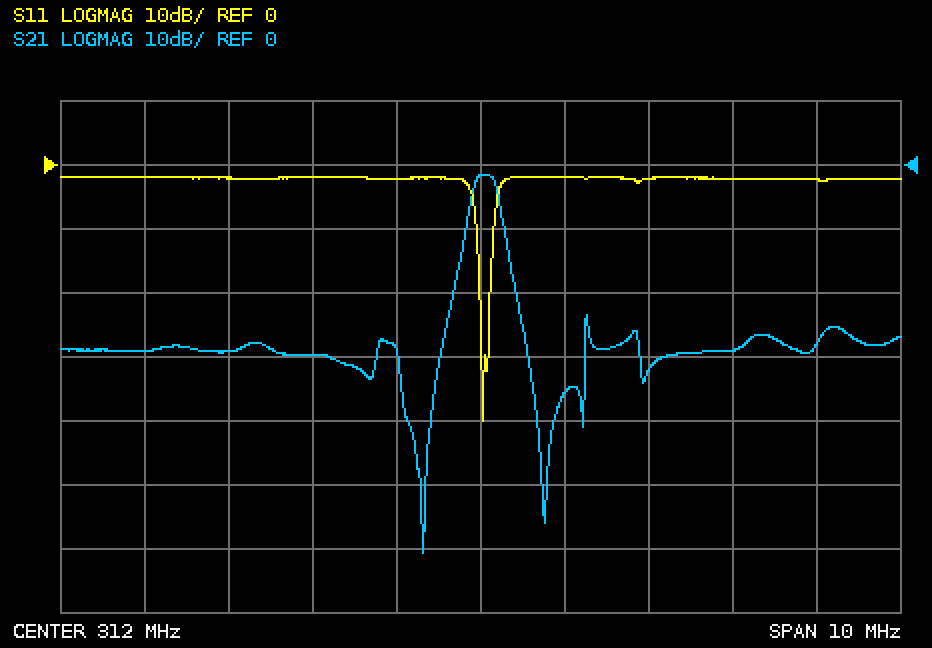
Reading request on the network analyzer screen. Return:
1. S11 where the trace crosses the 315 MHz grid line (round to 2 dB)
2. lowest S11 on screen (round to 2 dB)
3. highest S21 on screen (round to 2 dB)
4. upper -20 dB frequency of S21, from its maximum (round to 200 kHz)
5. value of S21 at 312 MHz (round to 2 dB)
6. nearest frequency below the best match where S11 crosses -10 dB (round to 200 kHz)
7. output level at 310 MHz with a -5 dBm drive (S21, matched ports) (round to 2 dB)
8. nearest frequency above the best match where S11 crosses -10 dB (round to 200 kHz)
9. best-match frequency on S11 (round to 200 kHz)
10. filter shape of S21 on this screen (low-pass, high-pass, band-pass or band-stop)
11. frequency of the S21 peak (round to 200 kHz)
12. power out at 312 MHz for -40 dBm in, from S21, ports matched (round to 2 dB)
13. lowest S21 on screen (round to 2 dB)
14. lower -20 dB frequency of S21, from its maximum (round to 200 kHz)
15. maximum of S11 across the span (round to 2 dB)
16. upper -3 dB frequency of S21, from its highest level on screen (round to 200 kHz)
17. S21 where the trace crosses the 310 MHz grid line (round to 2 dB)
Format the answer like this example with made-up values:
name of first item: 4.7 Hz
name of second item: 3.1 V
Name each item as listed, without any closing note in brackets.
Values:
S11 where the trace crosses the 315 MHz grid line: -2 dB
lowest S11 on screen: -40 dB
highest S21 on screen: -2 dB
upper -20 dB frequency of S21, from its maximum: 312.4 MHz
value of S21 at 312 MHz: -2 dB
nearest frequency below the best match where S11 crosses -10 dB: 312.0 MHz
output level at 310 MHz with a -5 dBm drive (S21, matched ports): -34 dBm
nearest frequency above the best match where S11 crosses -10 dB: 312.2 MHz
best-match frequency on S11: 312.0 MHz
filter shape of S21 on this screen: band-pass
frequency of the S21 peak: 312.0 MHz
power out at 312 MHz for -40 dBm in, from S21, ports matched: -42 dBm
lowest S21 on screen: -60 dB
lower -20 dB frequency of S21, from its maximum: 311.6 MHz
maximum of S11 across the span: -2 dB
upper -3 dB frequency of S21, from its highest level on screen: 312.2 MHz
S21 where the trace crosses the 310 MHz grid line: -30 dB
